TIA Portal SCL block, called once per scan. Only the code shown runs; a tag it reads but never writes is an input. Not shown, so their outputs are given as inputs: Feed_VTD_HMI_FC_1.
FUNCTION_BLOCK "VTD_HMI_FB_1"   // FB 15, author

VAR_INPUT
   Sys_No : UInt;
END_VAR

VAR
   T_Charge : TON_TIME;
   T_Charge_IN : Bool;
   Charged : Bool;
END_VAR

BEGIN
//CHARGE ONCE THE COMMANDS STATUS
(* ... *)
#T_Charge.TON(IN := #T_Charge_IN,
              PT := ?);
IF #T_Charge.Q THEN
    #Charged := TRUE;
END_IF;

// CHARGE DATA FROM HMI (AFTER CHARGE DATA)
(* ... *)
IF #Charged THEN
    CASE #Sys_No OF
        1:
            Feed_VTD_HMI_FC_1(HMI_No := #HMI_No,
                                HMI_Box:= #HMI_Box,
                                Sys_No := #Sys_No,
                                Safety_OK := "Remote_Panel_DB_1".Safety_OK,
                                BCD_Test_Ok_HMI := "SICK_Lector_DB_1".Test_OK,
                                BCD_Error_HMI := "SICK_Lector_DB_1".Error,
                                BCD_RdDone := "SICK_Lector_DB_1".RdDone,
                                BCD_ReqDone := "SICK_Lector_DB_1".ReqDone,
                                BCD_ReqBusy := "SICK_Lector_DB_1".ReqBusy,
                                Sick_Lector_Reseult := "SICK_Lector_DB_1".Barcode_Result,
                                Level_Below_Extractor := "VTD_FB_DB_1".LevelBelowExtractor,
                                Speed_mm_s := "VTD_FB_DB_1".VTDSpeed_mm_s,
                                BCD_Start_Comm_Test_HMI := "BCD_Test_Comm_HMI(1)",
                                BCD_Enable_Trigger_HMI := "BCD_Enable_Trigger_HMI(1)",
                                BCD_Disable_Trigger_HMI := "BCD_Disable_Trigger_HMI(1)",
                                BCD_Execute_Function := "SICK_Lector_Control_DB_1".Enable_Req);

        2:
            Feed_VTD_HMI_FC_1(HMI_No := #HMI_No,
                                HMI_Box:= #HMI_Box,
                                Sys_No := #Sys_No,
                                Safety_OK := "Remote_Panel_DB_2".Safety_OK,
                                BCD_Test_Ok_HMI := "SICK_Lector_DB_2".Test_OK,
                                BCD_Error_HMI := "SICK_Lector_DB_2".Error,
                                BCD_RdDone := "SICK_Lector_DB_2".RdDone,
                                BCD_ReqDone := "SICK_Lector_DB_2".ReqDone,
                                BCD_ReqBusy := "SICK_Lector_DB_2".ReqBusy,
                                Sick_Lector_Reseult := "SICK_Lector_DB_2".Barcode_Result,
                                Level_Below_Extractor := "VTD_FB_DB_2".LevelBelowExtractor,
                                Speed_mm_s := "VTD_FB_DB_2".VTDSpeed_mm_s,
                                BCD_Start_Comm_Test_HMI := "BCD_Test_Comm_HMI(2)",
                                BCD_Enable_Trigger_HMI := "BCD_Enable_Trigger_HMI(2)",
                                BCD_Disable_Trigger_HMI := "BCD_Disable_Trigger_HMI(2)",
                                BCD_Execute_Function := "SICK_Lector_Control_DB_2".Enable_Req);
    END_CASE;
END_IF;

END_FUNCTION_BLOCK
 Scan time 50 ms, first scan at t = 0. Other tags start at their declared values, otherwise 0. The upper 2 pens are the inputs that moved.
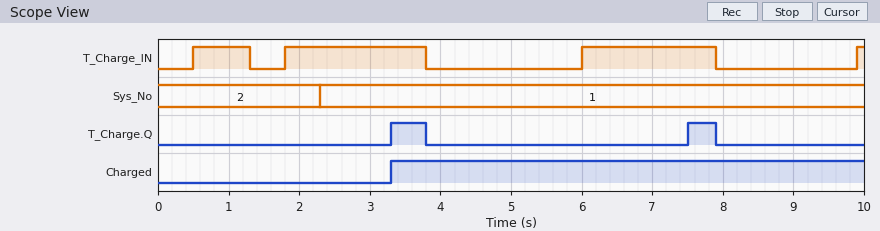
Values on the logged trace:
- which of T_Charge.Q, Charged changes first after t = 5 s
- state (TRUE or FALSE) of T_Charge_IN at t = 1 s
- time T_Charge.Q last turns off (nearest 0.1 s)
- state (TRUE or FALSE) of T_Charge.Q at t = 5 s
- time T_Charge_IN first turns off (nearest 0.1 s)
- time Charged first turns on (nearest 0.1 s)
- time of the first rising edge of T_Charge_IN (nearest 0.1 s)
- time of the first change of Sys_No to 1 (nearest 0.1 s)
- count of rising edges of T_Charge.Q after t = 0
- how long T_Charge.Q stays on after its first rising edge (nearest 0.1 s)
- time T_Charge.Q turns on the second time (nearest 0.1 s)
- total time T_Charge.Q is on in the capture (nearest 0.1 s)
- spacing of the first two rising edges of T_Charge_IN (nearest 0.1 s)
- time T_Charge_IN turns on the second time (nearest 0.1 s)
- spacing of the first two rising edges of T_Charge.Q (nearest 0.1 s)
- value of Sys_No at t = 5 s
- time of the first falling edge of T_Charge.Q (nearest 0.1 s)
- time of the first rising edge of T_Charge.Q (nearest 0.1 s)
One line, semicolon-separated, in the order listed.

T_Charge.Q; TRUE; 7.9 s; FALSE; 1.3 s; 3.3 s; 0.5 s; 2.3 s; 2; 0.5 s; 7.5 s; 0.9 s; 1.3 s; 1.8 s; 4.2 s; 1; 3.8 s; 3.3 s
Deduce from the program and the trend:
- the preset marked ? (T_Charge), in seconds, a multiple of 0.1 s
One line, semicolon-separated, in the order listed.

1.5 s
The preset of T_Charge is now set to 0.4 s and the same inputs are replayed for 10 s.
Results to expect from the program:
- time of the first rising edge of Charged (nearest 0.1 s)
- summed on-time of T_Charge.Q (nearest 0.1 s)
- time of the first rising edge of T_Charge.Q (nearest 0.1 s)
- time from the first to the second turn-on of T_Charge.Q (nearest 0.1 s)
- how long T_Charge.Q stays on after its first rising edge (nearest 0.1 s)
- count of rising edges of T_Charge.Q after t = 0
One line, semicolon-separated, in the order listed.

0.9 s; 3.5 s; 0.9 s; 1.3 s; 0.4 s; 3
